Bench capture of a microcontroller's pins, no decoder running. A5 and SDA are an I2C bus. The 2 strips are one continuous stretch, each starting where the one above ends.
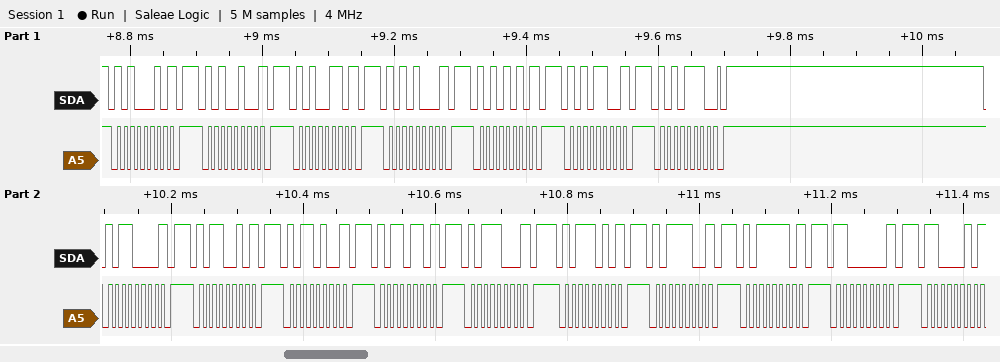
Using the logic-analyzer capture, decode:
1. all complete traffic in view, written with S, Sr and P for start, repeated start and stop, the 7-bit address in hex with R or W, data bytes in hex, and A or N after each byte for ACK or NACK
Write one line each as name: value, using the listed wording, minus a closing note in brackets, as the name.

all complete traffic in view, written with S, Sr and P for start, repeated start and stop, the 7-bit address in hex with R or W, data bytes in hex, and A or N after each byte for ACK or NACK: S 51W N P S 52W N P S 53W N P S 54W N P S 55W N P S 56W N P S 57W A P S 58W N P S 59W N P S 5AW N P S 5BW N P S 5CW N P S 5DW N P S 5EW N P S 5FW N P S 60W N P S 61W N
